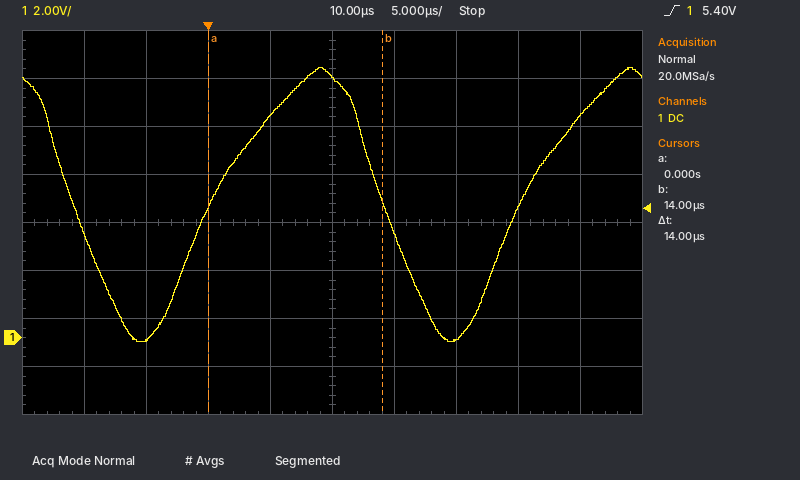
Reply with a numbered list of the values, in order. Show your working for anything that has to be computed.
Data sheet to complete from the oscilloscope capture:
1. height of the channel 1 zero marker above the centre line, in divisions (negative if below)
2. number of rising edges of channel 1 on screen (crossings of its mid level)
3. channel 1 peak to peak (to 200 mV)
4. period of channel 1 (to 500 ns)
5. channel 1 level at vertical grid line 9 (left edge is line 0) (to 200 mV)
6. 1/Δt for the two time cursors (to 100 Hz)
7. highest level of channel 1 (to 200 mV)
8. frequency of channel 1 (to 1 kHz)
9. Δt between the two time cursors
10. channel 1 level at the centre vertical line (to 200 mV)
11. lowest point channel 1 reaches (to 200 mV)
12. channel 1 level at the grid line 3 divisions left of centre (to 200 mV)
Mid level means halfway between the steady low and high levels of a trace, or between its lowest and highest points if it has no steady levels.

1. -2.4 div
2. 2
3. 11.2 V − (-200 mV) = 11.4 V
4. 25.0 µs
5. 9.2 V
6. 1 / 14 µs ≈ 71.4 kHz
7. 11.2 V
8. 1 / 25.0 µs ≈ 40 kHz
9. 14 µs
10. 10.8 V
11. -200 mV
12. 0.0 V
